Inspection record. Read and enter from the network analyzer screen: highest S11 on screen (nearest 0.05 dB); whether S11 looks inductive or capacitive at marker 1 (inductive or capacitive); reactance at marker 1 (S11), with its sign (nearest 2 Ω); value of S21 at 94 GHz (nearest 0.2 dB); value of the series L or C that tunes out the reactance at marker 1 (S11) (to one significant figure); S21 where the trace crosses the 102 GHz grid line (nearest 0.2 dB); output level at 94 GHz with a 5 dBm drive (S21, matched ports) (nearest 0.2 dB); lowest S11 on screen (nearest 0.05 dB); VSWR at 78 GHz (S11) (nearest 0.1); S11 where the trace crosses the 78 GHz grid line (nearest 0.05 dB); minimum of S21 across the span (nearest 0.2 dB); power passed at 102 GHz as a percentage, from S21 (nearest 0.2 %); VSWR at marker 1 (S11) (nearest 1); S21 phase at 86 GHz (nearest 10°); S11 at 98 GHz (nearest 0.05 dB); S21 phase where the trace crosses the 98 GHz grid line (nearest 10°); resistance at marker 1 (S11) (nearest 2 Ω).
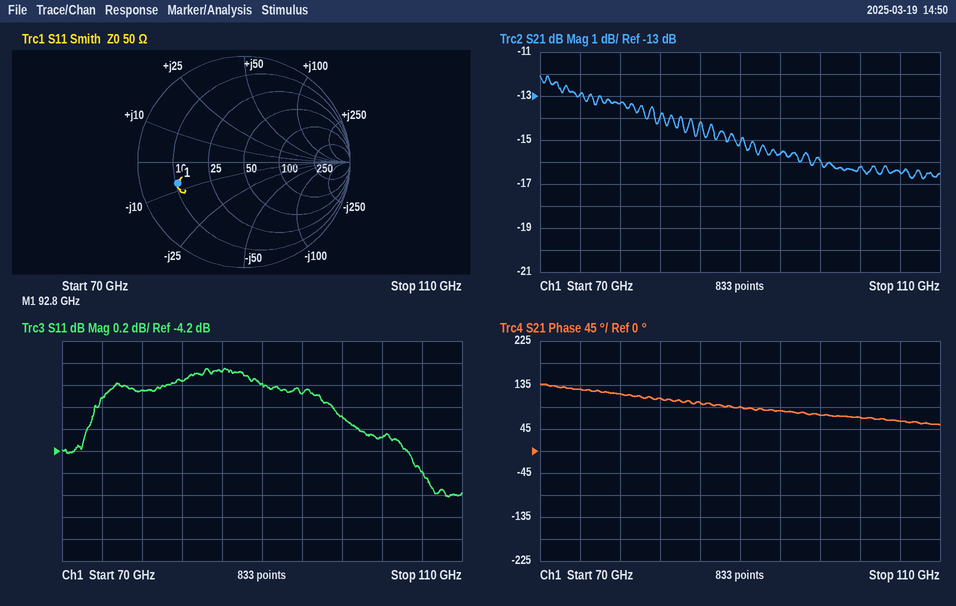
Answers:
-3.45 dB
capacitive
-8 Ω
-15.6 dB
10 pH
-16.2 dB
-10.6 dBm
-4.60 dB
4.8
-3.65 dB
-16.8 dB
2.4 %
5
100°
-3.90 dB
70°
10 Ω
